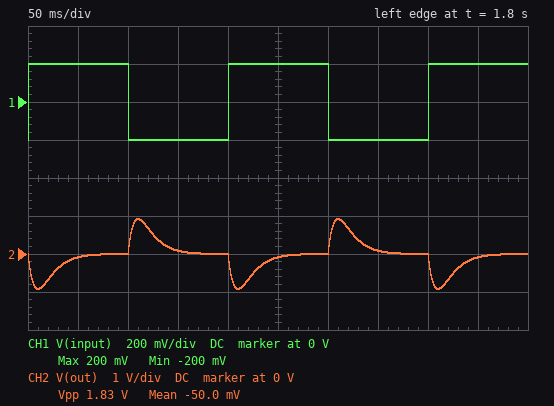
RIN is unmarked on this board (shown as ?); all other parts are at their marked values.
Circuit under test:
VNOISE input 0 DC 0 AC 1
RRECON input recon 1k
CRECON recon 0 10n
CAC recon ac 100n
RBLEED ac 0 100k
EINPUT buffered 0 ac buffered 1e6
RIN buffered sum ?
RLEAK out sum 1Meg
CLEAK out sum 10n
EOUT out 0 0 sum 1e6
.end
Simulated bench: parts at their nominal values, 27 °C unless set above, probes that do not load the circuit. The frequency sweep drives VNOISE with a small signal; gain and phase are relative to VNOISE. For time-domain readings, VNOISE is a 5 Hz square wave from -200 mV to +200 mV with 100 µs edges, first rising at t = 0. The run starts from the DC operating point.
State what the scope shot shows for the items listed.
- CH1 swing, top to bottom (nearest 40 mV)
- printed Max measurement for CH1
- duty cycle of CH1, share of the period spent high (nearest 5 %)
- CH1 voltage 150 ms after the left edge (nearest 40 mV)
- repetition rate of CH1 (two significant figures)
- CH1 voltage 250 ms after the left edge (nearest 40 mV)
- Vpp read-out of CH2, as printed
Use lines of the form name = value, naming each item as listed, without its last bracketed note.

CH1 swing, top to bottom = 400 mV
printed Max measurement for CH1 = 200 mV
duty cycle of CH1, share of the period spent high = 50 %
CH1 voltage 150 ms after the left edge = -200 mV
repetition rate of CH1 = 5.0 Hz
CH1 voltage 250 ms after the left edge = 200 mV
Vpp read-out of CH2, as printed = 1.83 V
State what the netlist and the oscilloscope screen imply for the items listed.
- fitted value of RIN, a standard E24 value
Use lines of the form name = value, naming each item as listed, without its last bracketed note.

fitted value of RIN, a standard E24 value = 160 kΩ
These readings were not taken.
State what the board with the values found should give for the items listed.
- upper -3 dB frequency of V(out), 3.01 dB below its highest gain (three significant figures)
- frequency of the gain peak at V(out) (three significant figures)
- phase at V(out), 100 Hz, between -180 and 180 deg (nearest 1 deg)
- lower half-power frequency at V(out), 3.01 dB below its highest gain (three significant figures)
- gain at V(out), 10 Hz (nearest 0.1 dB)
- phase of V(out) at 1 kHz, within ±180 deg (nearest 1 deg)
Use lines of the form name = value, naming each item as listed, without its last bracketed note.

upper -3 dB frequency of V(out), 3.01 dB below its highest gain = 38.2 Hz
frequency of the gain peak at V(out) = 15.8 Hz
phase at V(out), 100 Hz, between -180 and 180 deg = 108 deg
lower half-power frequency at V(out), 3.01 dB below its highest gain = 6.56 Hz
gain at V(out), 10 Hz = 9.0 dB
phase of V(out) at 1 kHz, within ±180 deg = 88 deg
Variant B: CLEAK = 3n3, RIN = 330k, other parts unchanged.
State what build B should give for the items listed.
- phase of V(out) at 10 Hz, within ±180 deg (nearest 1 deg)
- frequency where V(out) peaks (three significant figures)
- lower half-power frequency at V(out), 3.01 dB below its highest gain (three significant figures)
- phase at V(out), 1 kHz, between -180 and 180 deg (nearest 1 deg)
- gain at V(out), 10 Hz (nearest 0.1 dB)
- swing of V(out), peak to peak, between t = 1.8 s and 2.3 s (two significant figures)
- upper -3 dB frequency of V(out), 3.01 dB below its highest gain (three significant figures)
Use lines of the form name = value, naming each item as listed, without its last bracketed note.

phase of V(out) at 10 Hz, within ±180 deg = -134 deg
frequency where V(out) peaks = 27.6 Hz
lower half-power frequency at V(out), 3.01 dB below its highest gain = 10.2 Hz
phase at V(out), 1 kHz, between -180 and 180 deg = 90 deg
gain at V(out), 10 Hz = 3.9 dB
swing of V(out), peak to peak, between t = 1.8 s and 2.3 s = 1.4 V
upper -3 dB frequency of V(out), 3.01 dB below its highest gain = 74.2 Hz
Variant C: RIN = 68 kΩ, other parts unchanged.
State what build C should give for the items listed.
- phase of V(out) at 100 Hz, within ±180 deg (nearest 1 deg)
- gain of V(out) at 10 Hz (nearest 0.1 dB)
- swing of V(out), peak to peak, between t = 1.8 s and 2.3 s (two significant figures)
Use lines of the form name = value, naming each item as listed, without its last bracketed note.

phase of V(out) at 100 Hz, within ±180 deg = 108 deg
gain of V(out) at 10 Hz = 16.4 dB
swing of V(out), peak to peak, between t = 1.8 s and 2.3 s = 4.3 V
